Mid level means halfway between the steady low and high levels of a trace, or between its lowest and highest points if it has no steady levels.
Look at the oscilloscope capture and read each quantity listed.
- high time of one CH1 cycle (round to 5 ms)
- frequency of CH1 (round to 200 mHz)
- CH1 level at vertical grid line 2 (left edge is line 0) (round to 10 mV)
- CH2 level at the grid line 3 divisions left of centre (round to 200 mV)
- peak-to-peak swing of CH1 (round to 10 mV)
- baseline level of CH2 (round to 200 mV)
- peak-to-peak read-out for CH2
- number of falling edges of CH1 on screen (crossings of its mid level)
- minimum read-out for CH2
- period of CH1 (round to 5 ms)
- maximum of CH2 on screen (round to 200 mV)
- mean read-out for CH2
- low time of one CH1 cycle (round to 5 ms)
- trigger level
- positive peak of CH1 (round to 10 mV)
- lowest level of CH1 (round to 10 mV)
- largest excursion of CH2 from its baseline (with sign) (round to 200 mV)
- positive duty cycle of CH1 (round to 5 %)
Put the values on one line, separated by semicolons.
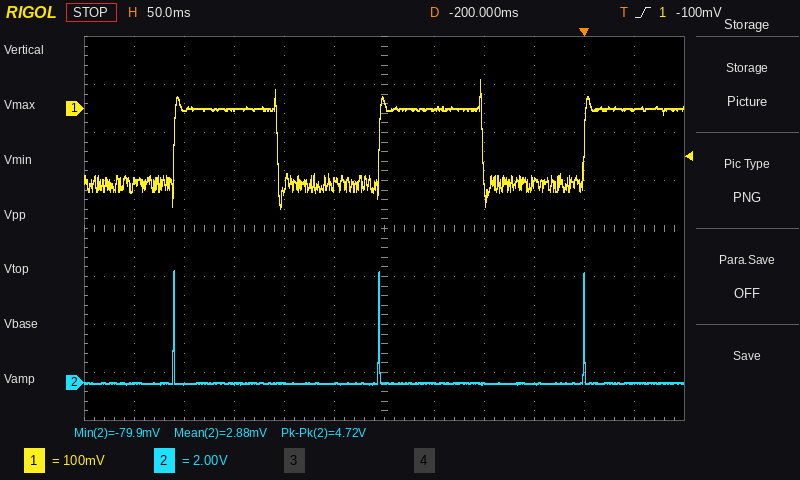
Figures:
105 ms; 4.8 Hz; 0 mV; 0.0 V; 270 mV; 0.0 V; 4.72 V; 2; -79.9 mV; 205 ms; 4.6 V; 2.88 mV; 100 ms; -100 mV; 60 mV; -210 mV; +4.6 V; 50 %
